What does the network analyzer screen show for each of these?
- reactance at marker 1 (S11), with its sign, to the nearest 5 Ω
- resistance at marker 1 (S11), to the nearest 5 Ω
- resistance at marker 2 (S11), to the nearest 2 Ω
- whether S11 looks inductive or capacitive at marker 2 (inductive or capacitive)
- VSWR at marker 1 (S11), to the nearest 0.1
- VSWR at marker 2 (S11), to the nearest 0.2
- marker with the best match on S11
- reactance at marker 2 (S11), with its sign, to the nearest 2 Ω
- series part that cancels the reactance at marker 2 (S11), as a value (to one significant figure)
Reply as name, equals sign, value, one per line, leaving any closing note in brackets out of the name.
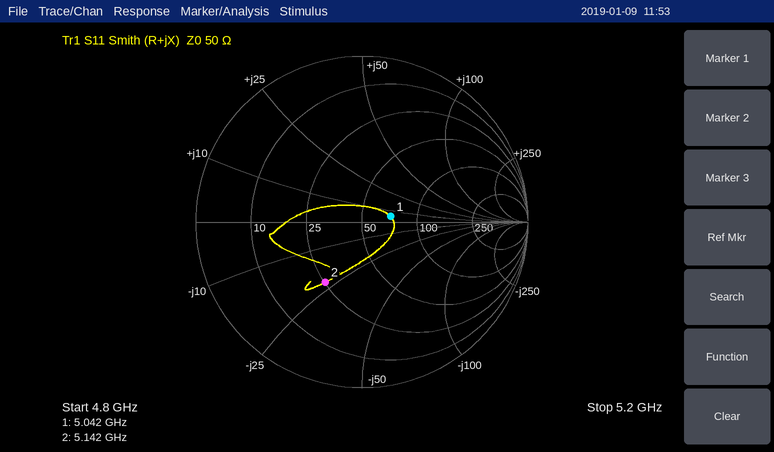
reactance at marker 1 (S11), with its sign, to the nearest 5 Ω = +5 Ω
resistance at marker 1 (S11), to the nearest 5 Ω = 70 Ω
resistance at marker 2 (S11), to the nearest 2 Ω = 26 Ω
whether S11 looks inductive or capacitive at marker 2 = capacitive
VSWR at marker 1 (S11), to the nearest 0.1 = 1.4
VSWR at marker 2 (S11), to the nearest 0.2 = 2.4
marker with the best match on S11 = marker 1
reactance at marker 2 (S11), with its sign, to the nearest 2 Ω = -22 Ω
series part that cancels the reactance at marker 2 (S11), as a value = 700 pH
